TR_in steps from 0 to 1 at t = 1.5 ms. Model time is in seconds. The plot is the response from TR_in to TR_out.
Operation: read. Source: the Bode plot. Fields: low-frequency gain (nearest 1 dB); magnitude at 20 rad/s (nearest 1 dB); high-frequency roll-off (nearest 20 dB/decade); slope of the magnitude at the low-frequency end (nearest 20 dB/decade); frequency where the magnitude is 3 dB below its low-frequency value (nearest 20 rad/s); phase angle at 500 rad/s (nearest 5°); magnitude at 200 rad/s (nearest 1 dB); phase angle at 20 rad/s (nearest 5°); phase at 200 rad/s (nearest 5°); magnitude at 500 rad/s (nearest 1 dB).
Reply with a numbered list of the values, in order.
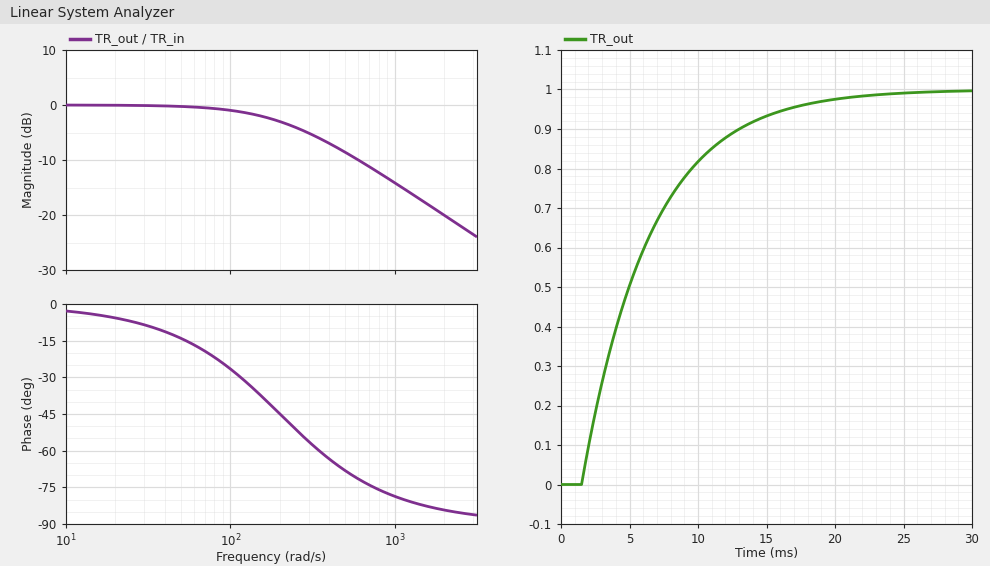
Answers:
1. 0 dB
2. 0 dB
3. -20 dB/decade
4. 0 dB/decade
5. 200 rad/s
6. -70°
7. -3 dB
8. -5°
9. -45°
10. -9 dB
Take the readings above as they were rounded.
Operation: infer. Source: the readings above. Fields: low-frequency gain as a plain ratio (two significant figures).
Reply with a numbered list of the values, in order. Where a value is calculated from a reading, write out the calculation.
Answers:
1. 10^(0 / 20) = 1.0
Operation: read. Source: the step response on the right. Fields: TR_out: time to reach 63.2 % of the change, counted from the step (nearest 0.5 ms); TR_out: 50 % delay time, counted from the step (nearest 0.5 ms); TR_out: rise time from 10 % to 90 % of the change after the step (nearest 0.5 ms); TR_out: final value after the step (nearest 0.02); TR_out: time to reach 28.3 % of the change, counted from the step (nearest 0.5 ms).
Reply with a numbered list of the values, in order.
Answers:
1. 5.0 ms
2. 3.5 ms
3. 11.0 ms
4. 1.00
5. 1.5 ms
